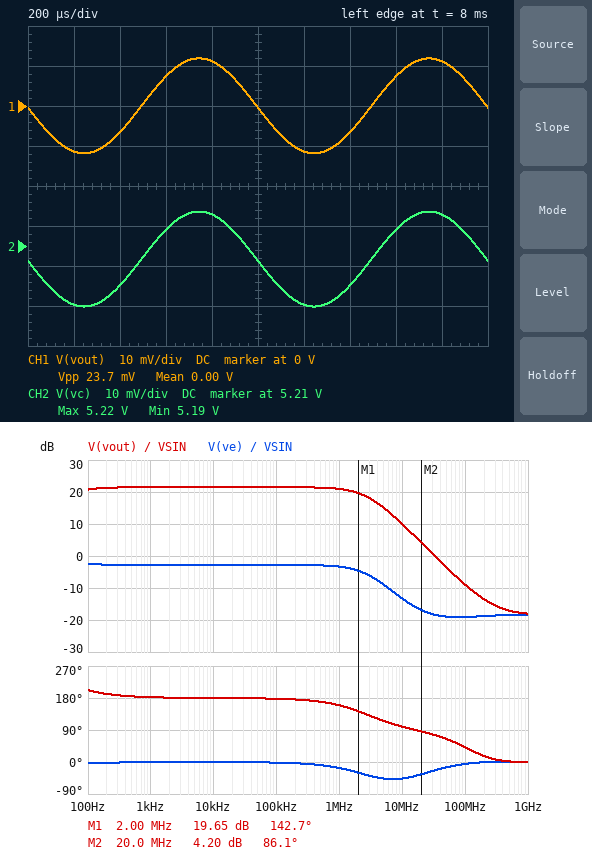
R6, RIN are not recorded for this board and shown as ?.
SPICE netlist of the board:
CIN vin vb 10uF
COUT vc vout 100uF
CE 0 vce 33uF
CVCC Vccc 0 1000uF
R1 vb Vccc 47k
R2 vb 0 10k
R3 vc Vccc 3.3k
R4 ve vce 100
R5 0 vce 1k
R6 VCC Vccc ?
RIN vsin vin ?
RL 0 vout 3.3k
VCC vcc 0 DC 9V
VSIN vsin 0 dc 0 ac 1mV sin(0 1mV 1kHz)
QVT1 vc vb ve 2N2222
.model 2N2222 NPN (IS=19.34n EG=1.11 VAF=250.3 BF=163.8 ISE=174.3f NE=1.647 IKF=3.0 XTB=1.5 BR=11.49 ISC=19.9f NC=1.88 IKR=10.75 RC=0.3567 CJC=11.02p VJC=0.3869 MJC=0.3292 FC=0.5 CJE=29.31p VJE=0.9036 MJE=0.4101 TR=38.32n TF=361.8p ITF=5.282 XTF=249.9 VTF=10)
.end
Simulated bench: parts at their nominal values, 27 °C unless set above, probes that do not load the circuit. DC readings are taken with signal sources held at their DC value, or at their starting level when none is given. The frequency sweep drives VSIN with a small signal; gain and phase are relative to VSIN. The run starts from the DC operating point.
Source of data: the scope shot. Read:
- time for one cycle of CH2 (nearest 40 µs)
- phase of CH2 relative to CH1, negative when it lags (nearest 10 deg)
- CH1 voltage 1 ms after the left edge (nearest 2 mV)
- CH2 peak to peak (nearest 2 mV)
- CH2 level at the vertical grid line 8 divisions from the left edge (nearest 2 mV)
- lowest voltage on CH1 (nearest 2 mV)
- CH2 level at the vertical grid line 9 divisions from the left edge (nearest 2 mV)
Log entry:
1.00 ms
0 deg
0 V
24 mV
5.214 V
-12 mV
5.218 V
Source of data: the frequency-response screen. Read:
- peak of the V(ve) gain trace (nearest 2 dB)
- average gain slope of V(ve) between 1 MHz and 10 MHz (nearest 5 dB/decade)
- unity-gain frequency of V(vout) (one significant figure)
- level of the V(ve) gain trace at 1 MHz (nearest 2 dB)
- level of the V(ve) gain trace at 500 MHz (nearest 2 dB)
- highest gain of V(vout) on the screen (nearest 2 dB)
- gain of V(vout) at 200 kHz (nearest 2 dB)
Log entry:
-2 dB
-10 dB/decade
30 MHz
-4 dB
-18 dB
22 dB
22 dB
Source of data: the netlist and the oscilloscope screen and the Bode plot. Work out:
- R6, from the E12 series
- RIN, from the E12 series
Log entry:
150 Ω
680 Ω
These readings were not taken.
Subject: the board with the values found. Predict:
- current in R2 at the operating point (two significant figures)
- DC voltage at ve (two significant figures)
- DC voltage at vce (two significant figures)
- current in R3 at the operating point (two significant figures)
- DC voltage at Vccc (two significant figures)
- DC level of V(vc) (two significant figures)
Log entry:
150 µA
1.2 V
1.1 V
1.1 mA
8.8 V
5.2 V
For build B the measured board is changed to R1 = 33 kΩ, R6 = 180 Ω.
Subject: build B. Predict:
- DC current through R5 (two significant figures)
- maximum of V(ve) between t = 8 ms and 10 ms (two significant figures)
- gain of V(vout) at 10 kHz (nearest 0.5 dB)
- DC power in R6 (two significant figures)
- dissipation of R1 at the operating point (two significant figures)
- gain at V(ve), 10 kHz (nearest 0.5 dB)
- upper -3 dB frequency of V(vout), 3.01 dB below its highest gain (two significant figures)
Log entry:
1.5 mA
1.7 V
22.0 dB
520 µW
1.4 mW
-2.5 dB
2.2 MHz
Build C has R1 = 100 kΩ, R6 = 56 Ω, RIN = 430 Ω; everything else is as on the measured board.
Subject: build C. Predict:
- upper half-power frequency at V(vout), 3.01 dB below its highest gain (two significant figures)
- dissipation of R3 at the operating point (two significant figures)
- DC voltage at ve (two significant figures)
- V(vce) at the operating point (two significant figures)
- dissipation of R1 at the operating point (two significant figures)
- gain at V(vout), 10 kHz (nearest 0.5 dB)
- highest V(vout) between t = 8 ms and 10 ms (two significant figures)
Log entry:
4.9 MHz
750 µW
530 mV
480 mV
670 µW
20.0 dB
10 mV
